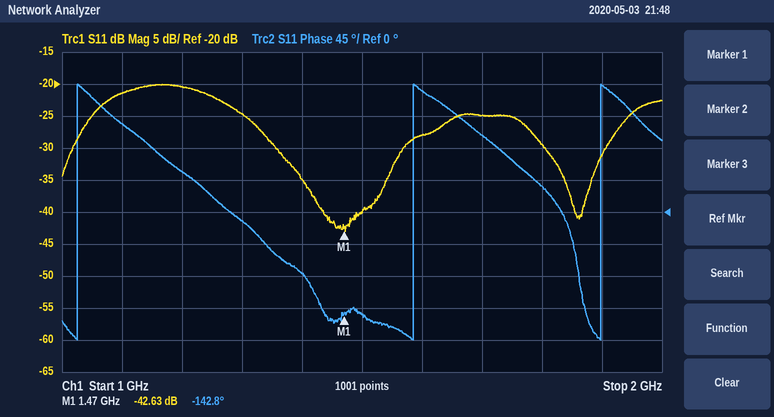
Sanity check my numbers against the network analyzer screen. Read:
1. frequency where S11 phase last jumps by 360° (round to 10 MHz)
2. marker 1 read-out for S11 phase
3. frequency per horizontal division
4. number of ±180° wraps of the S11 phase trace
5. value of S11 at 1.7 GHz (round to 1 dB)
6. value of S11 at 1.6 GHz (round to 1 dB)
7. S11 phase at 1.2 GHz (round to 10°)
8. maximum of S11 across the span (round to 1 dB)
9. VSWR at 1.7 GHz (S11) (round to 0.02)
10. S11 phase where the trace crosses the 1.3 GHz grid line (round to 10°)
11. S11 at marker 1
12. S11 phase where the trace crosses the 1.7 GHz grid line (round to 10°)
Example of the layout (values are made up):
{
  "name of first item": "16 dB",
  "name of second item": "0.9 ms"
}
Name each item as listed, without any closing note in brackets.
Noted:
{
  "frequency where S11 phase last jumps by 360°": "1.90 GHz",
  "marker 1 read-out for S11 phase": "-142.8°",
  "frequency per horizontal division": "100 MHz",
  "number of ±180° wraps of the S11 phase trace": "3",
  "value of S11 at 1.7 GHz": "-25 dB",
  "value of S11 at 1.6 GHz": "-28 dB",
  "S11 phase at 1.2 GHz": "60°",
  "maximum of S11 across the span": "-20 dB",
  "VSWR at 1.7 GHz (S11)": "1.12",
  "S11 phase where the trace crosses the 1.3 GHz grid line": "-10°",
  "S11 at marker 1": "-42.63 dB",
  "S11 phase where the trace crosses the 1.7 GHz grid line": "110°"
}
